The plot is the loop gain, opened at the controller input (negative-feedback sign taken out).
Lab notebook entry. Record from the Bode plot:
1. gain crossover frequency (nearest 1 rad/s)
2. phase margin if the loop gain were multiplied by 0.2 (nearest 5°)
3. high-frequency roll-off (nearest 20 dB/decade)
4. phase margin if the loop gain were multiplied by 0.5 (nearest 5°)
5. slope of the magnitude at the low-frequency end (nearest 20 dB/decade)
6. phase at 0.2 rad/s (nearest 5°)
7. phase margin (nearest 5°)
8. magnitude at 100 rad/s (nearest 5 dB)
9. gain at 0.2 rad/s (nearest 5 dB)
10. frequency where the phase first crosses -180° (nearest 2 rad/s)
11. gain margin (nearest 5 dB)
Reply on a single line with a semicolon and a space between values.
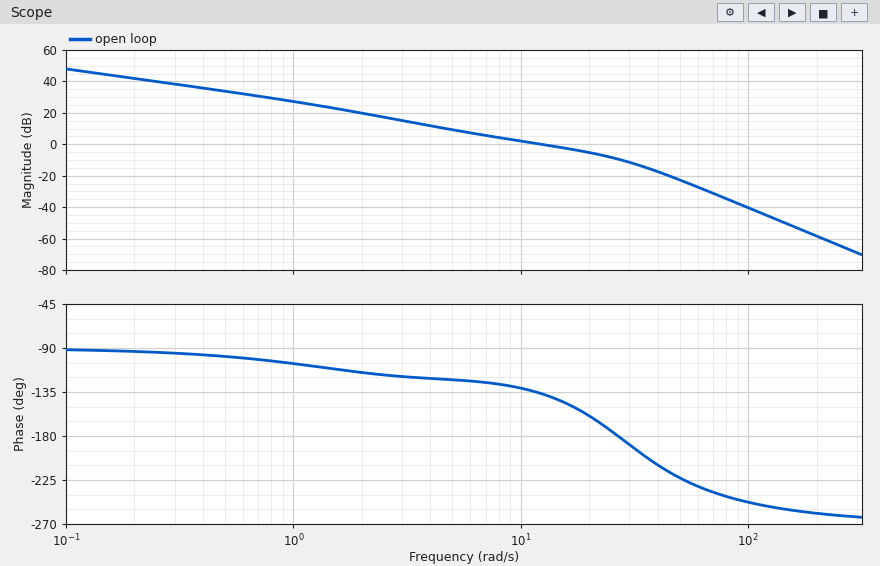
12 rad/s; 60°; -60 dB/decade; 55°; -20 dB/decade; -95°; 45°; -40 dB; 40 dB; 26 rad/s; 10 dB
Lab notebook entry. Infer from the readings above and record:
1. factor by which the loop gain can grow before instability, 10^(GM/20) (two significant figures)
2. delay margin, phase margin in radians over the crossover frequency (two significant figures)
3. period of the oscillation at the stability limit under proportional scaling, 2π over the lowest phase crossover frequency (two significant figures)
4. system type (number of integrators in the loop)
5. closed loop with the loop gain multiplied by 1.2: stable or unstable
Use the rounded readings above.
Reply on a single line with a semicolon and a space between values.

3.2; 0.065 s; 0.24 s; 1; stable
